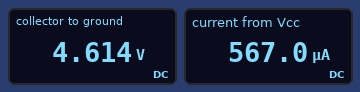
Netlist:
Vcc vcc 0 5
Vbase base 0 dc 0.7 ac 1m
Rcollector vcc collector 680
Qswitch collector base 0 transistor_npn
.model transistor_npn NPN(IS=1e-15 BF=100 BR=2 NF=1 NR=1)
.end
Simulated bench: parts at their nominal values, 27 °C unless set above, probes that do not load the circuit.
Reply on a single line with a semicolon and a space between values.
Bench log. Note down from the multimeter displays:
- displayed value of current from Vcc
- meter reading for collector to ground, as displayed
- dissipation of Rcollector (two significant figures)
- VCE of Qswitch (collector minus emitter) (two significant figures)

567.0 µA; 4.614 V; 220 µW; 4.6 V
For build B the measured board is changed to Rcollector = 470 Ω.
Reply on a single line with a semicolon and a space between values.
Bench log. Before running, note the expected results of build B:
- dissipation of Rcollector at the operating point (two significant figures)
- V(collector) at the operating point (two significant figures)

150 µW; 4.7 V
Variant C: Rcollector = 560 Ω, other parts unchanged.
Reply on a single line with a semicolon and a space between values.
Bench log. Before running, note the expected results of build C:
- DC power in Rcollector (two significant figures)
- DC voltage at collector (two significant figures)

180 µW; 4.7 V
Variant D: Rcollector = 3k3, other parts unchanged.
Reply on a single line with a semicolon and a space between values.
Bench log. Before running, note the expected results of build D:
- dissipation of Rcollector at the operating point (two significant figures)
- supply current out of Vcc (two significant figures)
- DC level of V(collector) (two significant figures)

1.1 mW; 570 µA; 3.1 V
